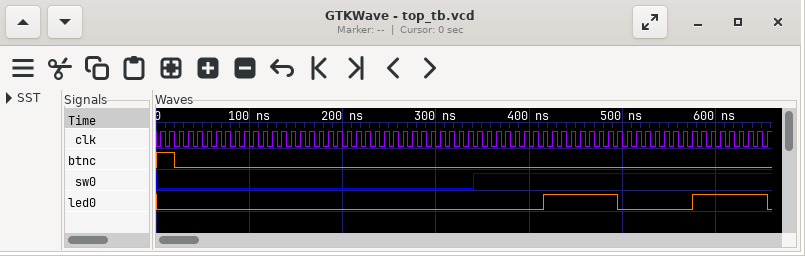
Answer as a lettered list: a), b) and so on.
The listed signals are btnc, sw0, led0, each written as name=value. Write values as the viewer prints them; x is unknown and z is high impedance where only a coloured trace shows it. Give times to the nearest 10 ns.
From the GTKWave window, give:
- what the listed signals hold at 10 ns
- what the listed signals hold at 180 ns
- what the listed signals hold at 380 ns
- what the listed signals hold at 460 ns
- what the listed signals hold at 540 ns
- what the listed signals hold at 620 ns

a) btnc=1, sw0=0, led0=0
b) btnc=0, sw0=0, led0=0
c) btnc=0, sw0=1, led0=0
d) btnc=0, sw0=1, led0=1
e) btnc=0, sw0=1, led0=0
f) btnc=0, sw0=1, led0=1
